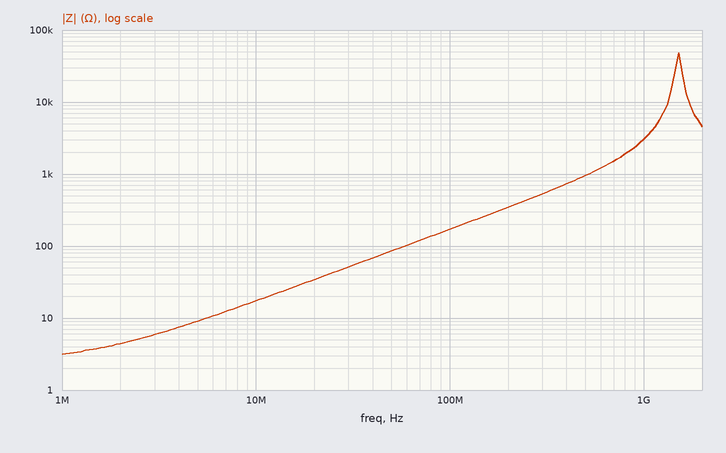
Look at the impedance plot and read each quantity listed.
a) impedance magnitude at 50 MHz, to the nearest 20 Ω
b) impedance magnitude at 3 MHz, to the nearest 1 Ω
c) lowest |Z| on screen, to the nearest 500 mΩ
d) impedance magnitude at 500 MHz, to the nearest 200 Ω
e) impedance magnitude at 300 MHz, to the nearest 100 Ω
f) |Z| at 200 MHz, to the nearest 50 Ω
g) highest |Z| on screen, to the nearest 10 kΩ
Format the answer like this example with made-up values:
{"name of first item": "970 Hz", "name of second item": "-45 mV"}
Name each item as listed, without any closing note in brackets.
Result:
{"impedance magnitude at 50 MHz, to the nearest 20 Ω": "80 Ω", "impedance magnitude at 3 MHz, to the nearest 1 Ω": "6 Ω", "lowest |Z| on screen, to the nearest 500 mΩ": "3.0 Ω", "impedance magnitude at 500 MHz, to the nearest 200 Ω": "1.0 kΩ", "impedance magnitude at 300 MHz, to the nearest 100 Ω": "500 Ω", "|Z| at 200 MHz, to the nearest 50 Ω": "350 Ω", "highest |Z| on screen, to the nearest 10 kΩ": "50 kΩ"}
